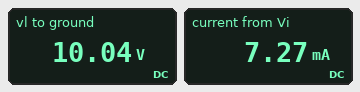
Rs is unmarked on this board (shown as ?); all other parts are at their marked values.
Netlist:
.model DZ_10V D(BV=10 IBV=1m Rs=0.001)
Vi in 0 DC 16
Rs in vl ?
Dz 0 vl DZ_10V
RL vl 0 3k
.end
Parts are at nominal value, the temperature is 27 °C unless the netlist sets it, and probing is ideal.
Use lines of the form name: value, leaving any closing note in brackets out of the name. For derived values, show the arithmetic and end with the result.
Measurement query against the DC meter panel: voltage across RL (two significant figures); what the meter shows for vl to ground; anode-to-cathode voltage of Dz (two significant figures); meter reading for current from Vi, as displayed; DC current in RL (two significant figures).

voltage across RL: 10.04 V = 10 V
what the meter shows for vl to ground: 10.04 V
anode-to-cathode voltage of Dz: 0 V - 10.04 V = -10 V
meter reading for current from Vi, as displayed: 7.27 mA
DC current in RL: (10.04 V) / 3 kΩ = 3.3 mA
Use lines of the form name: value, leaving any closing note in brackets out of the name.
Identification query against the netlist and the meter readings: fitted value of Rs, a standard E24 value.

fitted value of Rs, a standard E24 value: 820 Ω
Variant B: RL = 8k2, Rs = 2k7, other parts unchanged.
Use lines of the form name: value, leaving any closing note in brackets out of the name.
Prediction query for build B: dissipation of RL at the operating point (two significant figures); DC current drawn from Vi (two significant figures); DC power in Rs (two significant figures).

dissipation of RL at the operating point: 12 mW
DC current drawn from Vi: 2.2 mA
DC power in Rs: 13 mW
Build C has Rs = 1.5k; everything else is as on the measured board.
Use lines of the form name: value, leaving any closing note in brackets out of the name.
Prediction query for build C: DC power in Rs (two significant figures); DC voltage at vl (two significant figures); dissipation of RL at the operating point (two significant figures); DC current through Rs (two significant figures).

DC power in Rs: 24 mW
DC voltage at vl: 10 V
dissipation of RL at the operating point: 33 mW
DC current through Rs: 4.0 mA
